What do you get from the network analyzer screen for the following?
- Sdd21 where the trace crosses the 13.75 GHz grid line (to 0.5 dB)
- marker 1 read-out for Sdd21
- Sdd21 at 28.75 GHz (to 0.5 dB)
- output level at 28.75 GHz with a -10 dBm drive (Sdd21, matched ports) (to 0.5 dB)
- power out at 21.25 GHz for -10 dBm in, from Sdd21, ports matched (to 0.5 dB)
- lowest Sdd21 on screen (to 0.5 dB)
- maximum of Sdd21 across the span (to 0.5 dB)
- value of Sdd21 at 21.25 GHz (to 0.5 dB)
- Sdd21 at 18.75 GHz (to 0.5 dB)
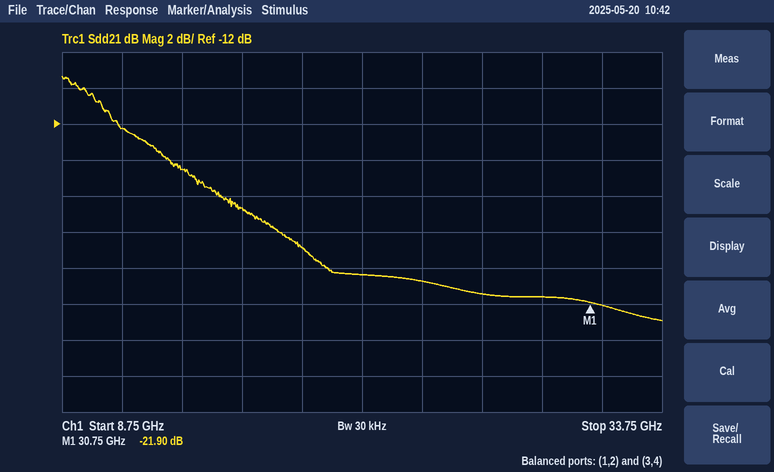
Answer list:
-14.5 dB
-21.90 dB
-21.5 dB
-31.5 dBm
-30.5 dBm
-23.0 dB
-9.5 dB
-20.5 dB
-19.0 dB
